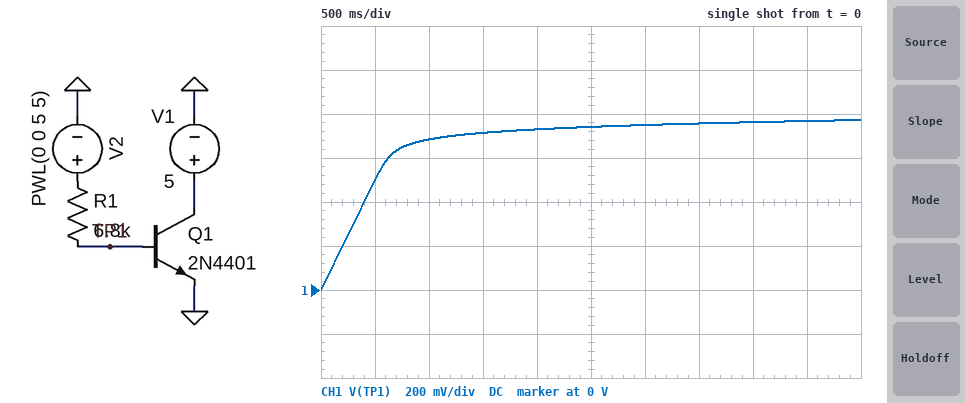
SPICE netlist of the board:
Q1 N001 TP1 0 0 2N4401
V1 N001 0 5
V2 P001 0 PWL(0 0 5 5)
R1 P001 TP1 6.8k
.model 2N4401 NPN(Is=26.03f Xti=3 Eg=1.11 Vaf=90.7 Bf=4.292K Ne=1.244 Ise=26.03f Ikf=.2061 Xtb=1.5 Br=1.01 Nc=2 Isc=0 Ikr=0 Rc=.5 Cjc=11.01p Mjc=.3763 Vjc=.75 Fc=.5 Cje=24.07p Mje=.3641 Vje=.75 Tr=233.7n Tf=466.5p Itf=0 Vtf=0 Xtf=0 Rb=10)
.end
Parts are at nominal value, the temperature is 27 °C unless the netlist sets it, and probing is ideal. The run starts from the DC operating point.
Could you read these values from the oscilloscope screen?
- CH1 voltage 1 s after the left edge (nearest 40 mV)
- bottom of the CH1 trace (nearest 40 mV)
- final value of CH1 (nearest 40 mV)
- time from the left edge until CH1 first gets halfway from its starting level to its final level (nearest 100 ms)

680 mV
0 V
760 mV
400 ms
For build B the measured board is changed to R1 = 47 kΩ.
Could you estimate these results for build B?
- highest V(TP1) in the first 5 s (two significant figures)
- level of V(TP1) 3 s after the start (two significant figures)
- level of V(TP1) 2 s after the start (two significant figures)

710 mV
690 mV
670 mV
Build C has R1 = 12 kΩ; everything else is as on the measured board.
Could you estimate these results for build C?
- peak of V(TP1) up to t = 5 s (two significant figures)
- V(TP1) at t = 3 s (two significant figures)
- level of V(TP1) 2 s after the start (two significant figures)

750 mV
730 mV
710 mV
